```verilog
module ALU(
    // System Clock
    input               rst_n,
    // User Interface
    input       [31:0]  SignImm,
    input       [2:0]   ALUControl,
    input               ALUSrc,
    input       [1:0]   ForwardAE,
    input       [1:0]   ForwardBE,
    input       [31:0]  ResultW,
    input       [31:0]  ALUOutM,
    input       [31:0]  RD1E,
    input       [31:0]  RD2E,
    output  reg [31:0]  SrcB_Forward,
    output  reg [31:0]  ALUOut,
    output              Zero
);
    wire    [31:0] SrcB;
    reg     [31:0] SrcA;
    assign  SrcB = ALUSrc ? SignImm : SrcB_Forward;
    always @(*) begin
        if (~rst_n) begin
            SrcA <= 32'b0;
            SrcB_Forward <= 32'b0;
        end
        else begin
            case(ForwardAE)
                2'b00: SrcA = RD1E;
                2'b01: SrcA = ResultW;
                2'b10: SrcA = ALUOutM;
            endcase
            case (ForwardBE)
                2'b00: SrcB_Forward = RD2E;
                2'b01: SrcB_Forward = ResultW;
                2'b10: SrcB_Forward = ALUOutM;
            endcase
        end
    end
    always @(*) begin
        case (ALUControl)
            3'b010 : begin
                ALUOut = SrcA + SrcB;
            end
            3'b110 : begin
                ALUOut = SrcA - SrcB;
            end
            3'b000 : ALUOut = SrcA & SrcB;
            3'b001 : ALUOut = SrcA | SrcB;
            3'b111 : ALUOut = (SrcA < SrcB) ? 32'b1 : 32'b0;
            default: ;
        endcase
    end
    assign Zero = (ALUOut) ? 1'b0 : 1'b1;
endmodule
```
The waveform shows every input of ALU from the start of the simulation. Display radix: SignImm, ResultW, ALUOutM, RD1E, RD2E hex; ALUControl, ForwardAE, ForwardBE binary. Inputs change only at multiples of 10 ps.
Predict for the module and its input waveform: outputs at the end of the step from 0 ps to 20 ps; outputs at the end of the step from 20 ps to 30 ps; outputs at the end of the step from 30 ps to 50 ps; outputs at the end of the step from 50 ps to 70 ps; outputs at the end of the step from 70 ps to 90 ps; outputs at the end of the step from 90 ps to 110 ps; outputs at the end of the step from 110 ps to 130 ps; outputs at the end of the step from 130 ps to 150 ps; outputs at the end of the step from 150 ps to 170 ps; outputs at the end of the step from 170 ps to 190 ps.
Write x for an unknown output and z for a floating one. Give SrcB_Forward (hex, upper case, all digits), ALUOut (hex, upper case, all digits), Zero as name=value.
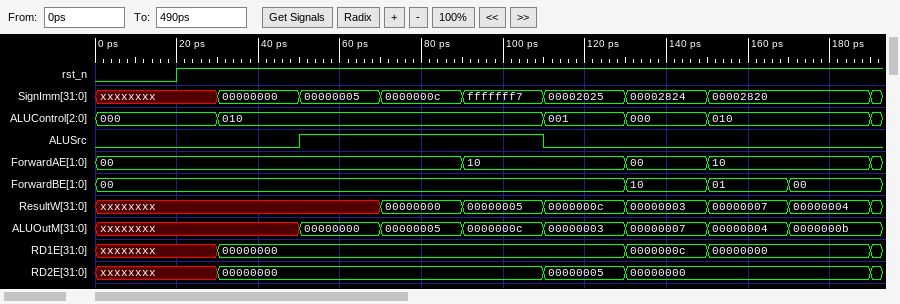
SrcB_Forward=00000000, ALUOut=00000000, Zero=1
SrcB_Forward=x, ALUOut=x, Zero=x
SrcB_Forward=00000000, ALUOut=00000000, Zero=1
SrcB_Forward=00000000, ALUOut=00000005, Zero=0
SrcB_Forward=00000000, ALUOut=0000000C, Zero=0
SrcB_Forward=00000000, ALUOut=00000003, Zero=0
SrcB_Forward=00000005, ALUOut=00000007, Zero=0
SrcB_Forward=00000007, ALUOut=00000004, Zero=0
SrcB_Forward=00000007, ALUOut=0000000B, Zero=0
SrcB_Forward=00000000, ALUOut=0000000B, Zero=0
